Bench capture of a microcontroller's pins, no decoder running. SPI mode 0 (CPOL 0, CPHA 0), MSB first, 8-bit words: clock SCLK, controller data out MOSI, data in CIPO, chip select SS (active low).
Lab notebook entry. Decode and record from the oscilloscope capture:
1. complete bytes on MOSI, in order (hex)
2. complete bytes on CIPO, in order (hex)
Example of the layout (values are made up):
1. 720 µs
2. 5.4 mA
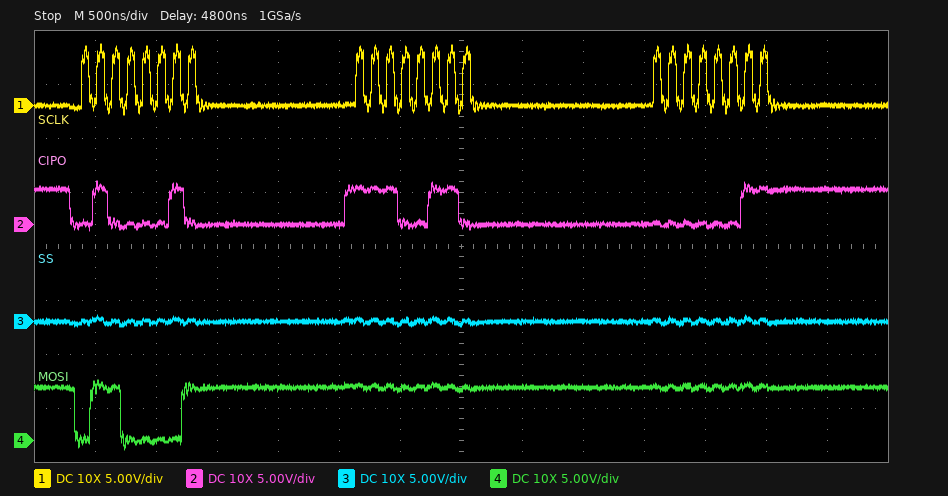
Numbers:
1. 61 FF FF
2. 42 E6 03
